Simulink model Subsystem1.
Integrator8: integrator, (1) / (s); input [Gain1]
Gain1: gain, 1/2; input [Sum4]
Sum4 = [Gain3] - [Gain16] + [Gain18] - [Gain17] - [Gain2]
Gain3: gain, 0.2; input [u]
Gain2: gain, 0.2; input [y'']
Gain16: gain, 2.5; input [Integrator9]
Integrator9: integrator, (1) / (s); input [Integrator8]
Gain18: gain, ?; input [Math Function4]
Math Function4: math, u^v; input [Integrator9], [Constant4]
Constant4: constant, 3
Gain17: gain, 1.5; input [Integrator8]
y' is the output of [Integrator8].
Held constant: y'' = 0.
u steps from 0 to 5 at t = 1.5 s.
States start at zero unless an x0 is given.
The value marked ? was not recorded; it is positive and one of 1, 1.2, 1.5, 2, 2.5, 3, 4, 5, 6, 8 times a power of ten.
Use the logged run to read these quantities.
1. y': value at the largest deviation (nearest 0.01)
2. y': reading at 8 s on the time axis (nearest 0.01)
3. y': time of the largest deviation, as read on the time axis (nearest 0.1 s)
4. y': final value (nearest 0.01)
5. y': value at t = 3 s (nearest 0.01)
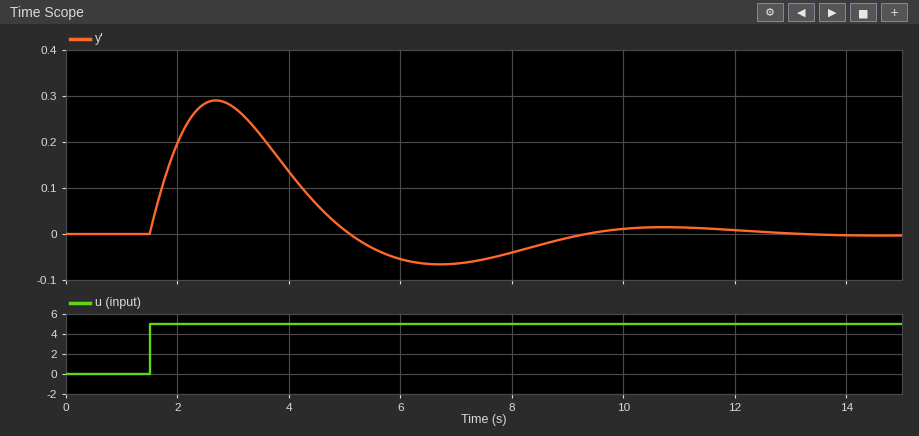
0.29
-0.04
2.7 s
0.00
0.28
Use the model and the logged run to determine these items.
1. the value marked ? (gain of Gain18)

1.5
